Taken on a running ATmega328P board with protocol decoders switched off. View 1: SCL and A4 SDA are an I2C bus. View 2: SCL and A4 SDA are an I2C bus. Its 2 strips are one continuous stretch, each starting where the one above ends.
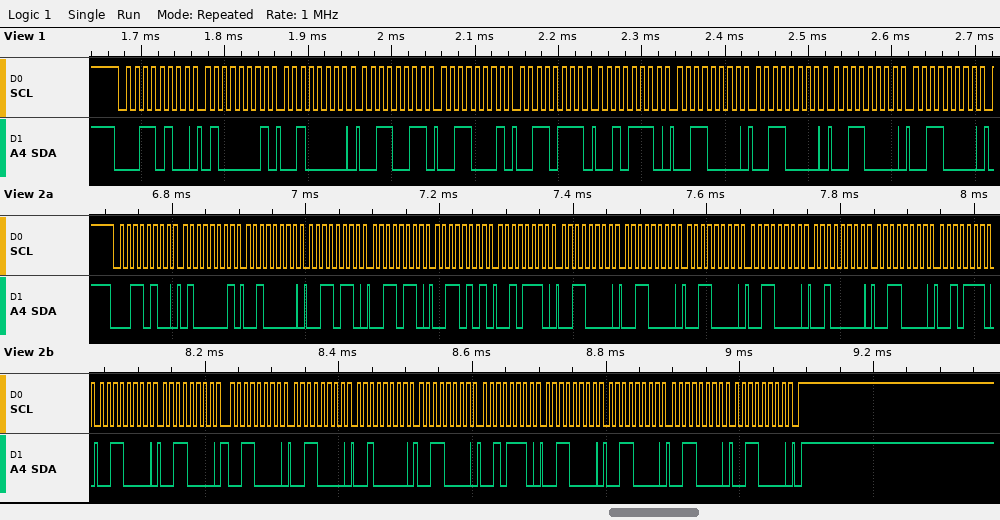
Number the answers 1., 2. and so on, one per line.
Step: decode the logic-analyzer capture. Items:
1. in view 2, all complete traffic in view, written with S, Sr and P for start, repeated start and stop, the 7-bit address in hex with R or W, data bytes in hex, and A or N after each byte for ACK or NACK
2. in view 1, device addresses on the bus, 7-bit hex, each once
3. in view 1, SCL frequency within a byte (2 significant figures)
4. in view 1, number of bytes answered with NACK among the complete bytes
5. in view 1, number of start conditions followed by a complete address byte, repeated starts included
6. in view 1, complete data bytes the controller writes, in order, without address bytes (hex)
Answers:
1. S 1AW A 41 A 20 A 36 A 36 A 35 A 2E A 30 A 30 A 30 A 30 A 20 A 30 A 2E A 30 A 30 A 30 A 30 A 20 A 30 A 2E A 30 A 30 A 30 A 30 A P
2. 0x1A
3. 100 kHz
4. 0
5. 1
6. 41 20 33 31 37 2E 30 30 30 30
